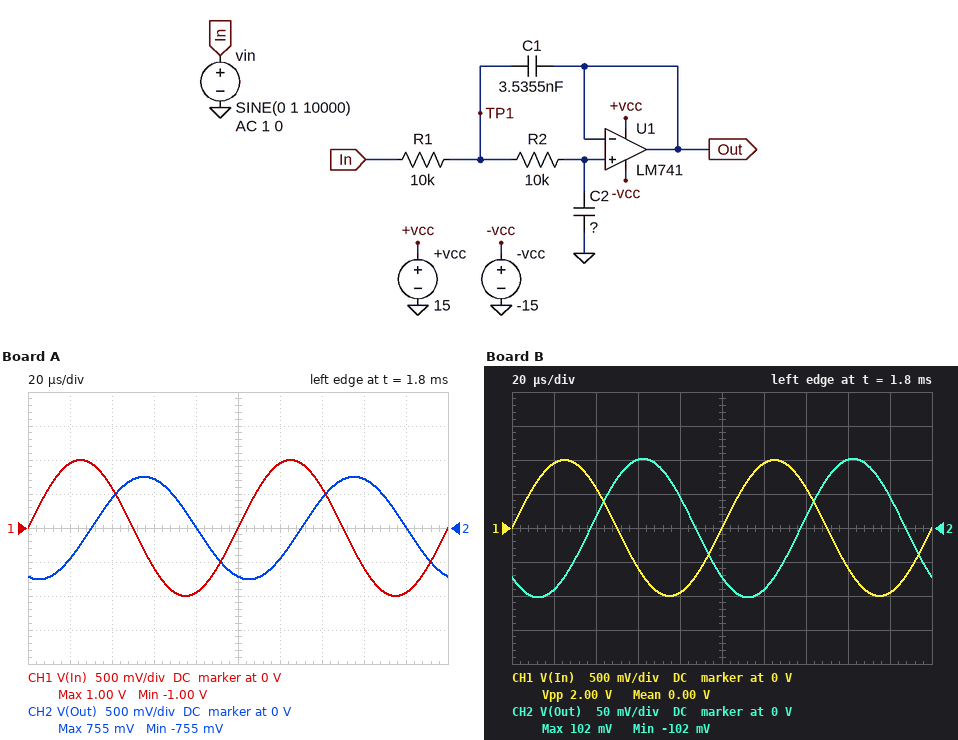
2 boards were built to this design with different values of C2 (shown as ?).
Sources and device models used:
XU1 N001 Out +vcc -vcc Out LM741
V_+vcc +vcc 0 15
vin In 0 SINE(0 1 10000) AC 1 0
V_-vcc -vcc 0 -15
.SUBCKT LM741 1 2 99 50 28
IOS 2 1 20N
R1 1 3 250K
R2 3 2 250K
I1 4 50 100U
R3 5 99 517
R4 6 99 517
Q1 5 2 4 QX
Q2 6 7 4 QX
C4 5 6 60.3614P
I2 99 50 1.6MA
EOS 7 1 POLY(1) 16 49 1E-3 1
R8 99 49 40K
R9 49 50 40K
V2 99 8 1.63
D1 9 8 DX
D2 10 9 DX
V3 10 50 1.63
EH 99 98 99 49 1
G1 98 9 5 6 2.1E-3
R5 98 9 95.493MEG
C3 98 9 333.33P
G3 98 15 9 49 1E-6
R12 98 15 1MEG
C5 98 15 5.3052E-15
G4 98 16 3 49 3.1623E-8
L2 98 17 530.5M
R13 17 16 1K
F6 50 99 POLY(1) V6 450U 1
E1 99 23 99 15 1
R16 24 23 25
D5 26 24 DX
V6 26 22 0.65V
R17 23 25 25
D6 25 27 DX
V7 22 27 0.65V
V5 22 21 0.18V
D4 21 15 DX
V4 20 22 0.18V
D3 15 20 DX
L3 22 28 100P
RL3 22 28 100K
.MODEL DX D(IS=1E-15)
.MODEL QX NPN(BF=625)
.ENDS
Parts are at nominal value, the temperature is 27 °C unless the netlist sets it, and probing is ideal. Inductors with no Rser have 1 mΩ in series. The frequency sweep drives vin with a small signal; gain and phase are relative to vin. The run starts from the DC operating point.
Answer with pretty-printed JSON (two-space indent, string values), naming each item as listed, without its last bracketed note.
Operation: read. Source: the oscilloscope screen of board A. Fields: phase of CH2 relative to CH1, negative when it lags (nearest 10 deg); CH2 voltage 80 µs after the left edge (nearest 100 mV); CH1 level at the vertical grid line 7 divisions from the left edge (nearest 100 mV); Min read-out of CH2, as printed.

{
  "phase of CH2 relative to CH1, negative when it lags": "-110 deg",
  "CH2 voltage 80 µs after the left edge": "0 V",
  "CH1 level at the vertical grid line 7 divisions from the left edge": "600 mV",
  "Min read-out of CH2, as printed": "-755 mV"
}
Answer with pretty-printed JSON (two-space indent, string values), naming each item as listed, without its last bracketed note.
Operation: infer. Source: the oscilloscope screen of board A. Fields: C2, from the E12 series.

{
  "C2, from the E12 series": "1 nF"
}
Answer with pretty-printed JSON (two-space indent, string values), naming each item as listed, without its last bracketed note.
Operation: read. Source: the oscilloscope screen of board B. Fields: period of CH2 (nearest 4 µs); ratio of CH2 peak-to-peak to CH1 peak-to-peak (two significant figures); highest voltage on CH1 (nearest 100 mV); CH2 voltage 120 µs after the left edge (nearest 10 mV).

{
  "period of CH2": "100 µs",
  "ratio of CH2 peak-to-peak to CH1 peak-to-peak": "0.10",
  "highest voltage on CH1": "1.0 V",
  "CH2 voltage 120 µs after the left edge": "-90 mV"
}
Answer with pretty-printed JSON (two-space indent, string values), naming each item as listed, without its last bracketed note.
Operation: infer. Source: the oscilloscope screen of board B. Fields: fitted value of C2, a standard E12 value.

{
  "fitted value of C2, a standard E12 value": "5.6 nF"
}
